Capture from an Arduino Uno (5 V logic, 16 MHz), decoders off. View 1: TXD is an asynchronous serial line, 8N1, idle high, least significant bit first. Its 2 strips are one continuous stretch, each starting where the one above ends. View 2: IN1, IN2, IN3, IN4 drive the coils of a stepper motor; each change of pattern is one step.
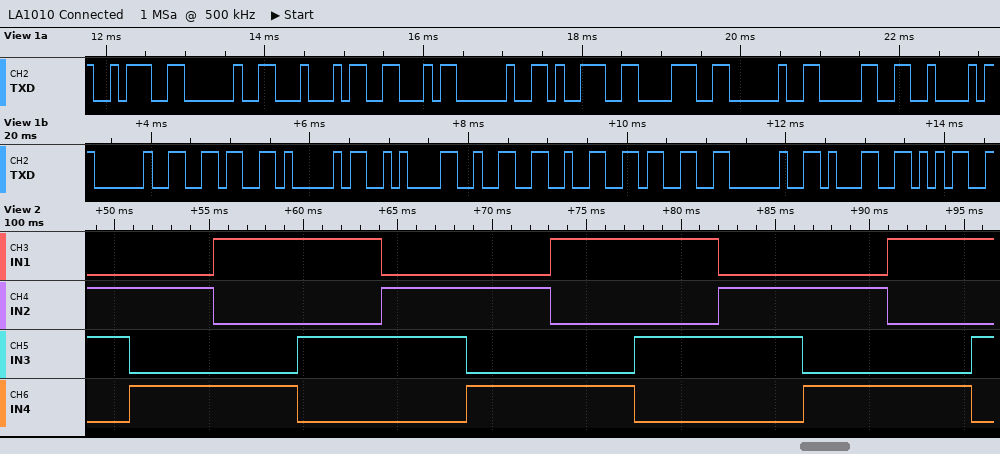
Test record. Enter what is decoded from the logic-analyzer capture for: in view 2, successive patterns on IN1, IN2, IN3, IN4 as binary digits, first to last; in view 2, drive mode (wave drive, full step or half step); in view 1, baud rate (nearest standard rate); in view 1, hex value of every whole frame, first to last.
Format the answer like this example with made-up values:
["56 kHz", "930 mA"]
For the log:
["0110 0101 1001 1010 0110 0101 1001 1010 0110 0101 1001 1010", "full step", "9600 baud", "3A 20 44 46 20 39 38 20 30 42 20 36 41 0A 32 32 33 20 31 35"]
